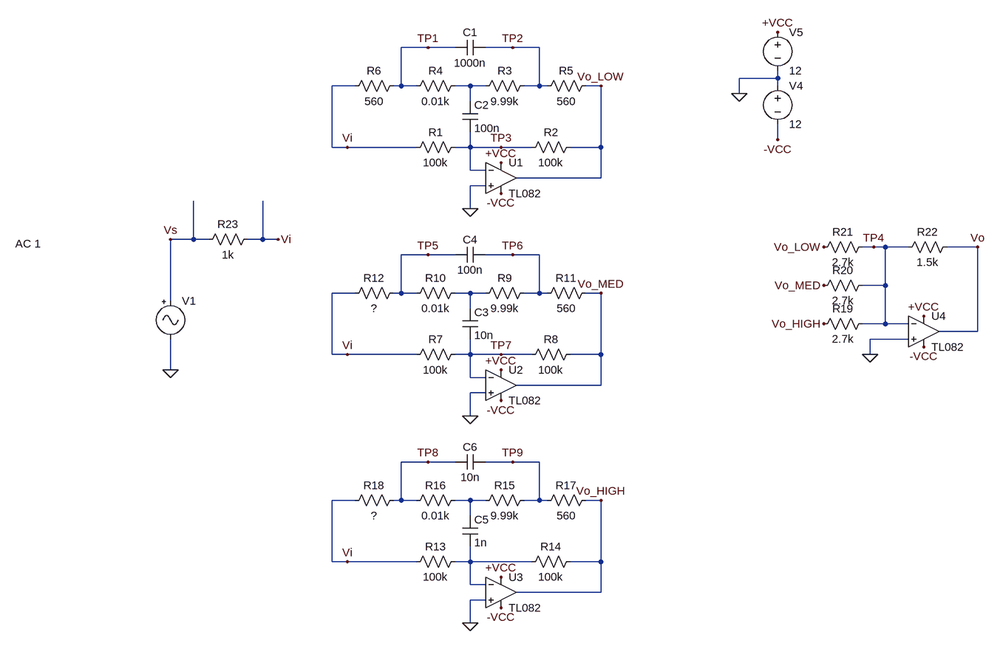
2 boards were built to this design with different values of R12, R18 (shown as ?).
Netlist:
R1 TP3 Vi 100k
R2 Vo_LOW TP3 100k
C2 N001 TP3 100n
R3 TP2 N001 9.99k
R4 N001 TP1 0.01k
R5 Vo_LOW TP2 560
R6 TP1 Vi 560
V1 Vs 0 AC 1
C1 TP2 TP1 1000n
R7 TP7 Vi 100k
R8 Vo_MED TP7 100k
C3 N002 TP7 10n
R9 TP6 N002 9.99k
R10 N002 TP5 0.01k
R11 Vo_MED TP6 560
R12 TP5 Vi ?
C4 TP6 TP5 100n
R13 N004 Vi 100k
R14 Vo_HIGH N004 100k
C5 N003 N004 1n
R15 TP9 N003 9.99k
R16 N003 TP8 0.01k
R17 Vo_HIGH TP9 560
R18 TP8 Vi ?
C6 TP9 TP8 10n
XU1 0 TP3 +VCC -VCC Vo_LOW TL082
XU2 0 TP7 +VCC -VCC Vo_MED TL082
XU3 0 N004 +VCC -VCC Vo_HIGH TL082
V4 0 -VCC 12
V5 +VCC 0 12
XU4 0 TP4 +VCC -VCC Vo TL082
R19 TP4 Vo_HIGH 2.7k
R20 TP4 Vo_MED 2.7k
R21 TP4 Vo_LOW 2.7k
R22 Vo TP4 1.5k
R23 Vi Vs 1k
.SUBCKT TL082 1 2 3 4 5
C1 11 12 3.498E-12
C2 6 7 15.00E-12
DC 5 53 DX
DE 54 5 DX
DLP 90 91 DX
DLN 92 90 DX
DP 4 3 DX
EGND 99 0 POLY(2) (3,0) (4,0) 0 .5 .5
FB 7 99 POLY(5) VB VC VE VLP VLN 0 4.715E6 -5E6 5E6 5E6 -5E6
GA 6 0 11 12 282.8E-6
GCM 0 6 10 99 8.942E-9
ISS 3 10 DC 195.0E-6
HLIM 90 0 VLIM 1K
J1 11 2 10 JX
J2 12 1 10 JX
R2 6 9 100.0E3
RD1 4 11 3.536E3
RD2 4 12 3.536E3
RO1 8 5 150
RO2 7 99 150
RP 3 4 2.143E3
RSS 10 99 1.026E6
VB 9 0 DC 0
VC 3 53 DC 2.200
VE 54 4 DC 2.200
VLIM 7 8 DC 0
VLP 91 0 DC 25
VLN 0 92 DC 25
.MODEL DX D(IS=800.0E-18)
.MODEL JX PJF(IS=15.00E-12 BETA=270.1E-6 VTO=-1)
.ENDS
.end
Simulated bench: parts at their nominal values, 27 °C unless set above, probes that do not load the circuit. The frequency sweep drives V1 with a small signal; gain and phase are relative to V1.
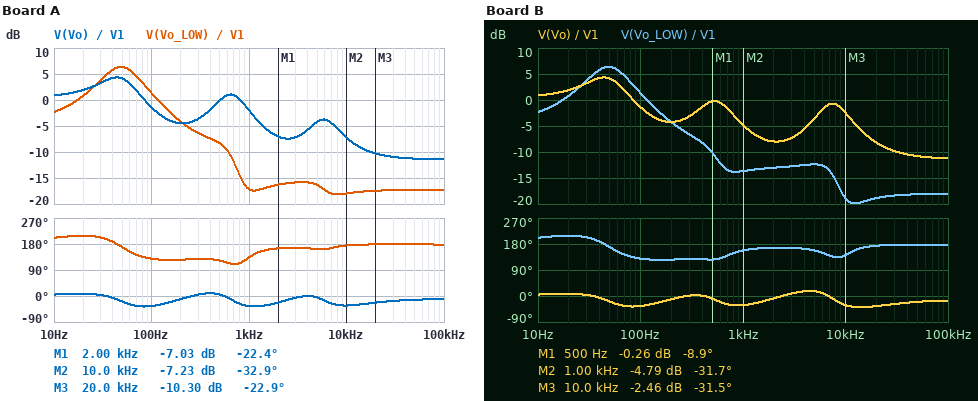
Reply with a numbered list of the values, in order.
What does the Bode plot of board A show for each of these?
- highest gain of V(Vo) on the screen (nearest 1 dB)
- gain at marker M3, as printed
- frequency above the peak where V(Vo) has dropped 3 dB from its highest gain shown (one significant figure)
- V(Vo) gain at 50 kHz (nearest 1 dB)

1. 4 dB
2. -10.30 dB
3. 70 Hz
4. -11 dB
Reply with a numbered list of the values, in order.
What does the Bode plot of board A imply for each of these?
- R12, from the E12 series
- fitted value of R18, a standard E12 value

1. 330 Ω
2. 680 Ω
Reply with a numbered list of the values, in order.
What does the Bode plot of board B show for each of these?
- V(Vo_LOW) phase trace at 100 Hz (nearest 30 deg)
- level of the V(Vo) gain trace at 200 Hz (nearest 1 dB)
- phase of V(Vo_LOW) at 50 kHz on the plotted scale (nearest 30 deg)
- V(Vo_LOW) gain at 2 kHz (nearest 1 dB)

1. 120 deg
2. -4 dB
3. 180 deg
4. -13 dB
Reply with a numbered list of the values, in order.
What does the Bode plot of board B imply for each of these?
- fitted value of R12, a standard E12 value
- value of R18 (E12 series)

1. 680 Ω
2. 270 Ω
